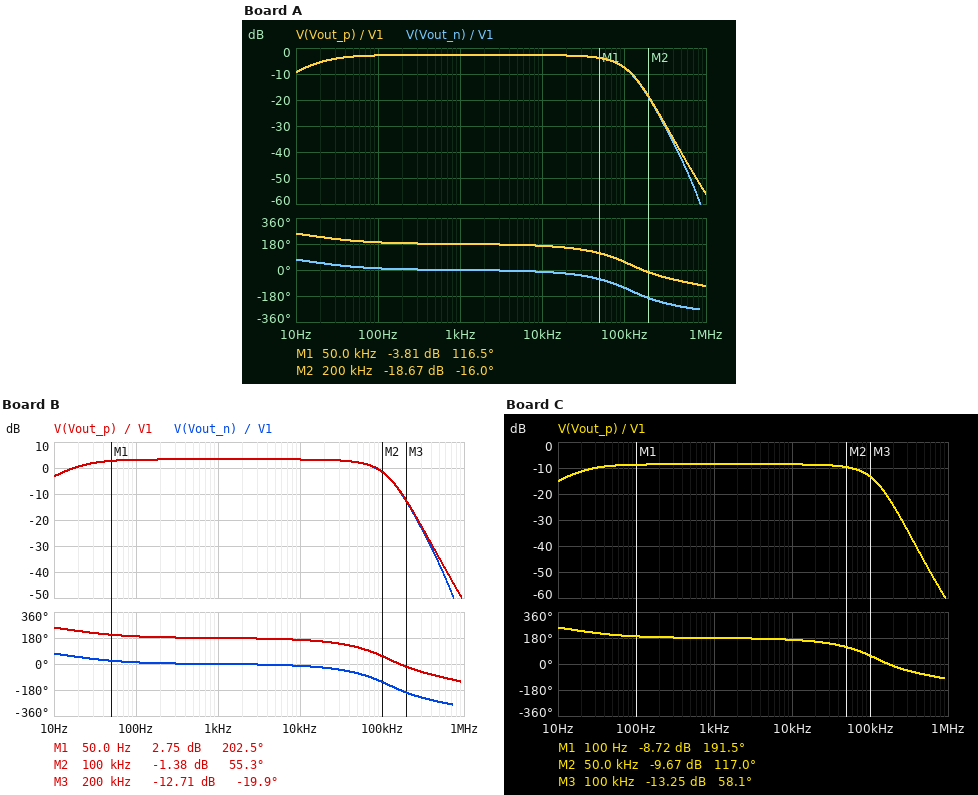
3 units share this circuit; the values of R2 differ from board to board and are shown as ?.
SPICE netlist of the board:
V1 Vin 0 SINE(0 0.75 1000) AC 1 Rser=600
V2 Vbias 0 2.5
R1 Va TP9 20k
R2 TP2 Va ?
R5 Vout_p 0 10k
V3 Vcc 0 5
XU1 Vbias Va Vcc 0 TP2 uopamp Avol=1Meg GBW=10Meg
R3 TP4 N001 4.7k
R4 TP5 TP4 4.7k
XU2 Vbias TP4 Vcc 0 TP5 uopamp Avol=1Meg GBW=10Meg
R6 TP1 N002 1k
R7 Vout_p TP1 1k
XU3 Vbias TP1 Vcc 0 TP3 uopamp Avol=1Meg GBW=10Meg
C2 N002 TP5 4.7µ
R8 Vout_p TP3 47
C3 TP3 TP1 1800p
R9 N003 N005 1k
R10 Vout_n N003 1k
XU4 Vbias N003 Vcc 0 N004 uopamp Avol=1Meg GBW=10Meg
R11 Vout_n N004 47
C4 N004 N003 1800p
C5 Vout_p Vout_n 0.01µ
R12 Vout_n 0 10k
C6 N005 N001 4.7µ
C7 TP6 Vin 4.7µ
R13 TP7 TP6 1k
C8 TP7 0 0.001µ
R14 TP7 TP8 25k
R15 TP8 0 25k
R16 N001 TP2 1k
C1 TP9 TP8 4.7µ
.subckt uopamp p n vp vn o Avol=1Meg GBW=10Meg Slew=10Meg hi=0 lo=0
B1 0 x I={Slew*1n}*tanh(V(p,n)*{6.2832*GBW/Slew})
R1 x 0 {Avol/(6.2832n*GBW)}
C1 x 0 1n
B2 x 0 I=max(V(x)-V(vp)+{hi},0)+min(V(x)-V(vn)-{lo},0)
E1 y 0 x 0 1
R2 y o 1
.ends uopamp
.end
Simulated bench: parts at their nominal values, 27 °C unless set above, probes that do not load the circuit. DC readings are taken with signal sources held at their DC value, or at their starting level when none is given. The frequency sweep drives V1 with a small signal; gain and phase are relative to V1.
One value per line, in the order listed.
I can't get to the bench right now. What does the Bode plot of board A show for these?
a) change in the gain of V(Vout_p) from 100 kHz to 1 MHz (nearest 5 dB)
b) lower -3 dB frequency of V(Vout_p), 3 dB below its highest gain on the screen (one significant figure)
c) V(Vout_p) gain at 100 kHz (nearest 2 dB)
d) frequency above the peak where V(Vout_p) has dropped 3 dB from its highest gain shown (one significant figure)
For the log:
-50 dB
20 Hz
-8 dB
80 kHz
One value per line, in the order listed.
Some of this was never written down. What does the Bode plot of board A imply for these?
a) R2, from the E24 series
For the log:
110 kΩ
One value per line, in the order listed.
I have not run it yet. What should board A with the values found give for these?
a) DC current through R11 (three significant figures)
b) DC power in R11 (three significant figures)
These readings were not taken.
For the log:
250 µA
2.94 µW
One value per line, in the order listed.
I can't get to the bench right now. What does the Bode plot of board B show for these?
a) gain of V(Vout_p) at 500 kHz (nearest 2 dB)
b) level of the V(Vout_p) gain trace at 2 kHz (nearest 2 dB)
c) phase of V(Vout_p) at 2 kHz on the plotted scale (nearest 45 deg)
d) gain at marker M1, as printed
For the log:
-34 dB
4 dB
180 deg
2.75 dB
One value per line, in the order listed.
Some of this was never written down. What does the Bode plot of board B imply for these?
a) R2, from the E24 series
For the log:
220 kΩ
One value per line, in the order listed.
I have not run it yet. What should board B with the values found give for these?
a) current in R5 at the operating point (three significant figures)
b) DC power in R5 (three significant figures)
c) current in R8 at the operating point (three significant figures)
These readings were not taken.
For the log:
250 µA
625 µW
250 µA
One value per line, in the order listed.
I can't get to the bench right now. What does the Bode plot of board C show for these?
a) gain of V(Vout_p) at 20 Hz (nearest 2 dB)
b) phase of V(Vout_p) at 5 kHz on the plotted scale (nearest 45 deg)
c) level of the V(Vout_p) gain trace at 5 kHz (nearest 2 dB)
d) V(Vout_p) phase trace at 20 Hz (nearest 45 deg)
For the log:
-12 dB
180 deg
-8 dB
225 deg
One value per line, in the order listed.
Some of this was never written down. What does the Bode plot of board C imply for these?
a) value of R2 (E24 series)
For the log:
56 kΩ
